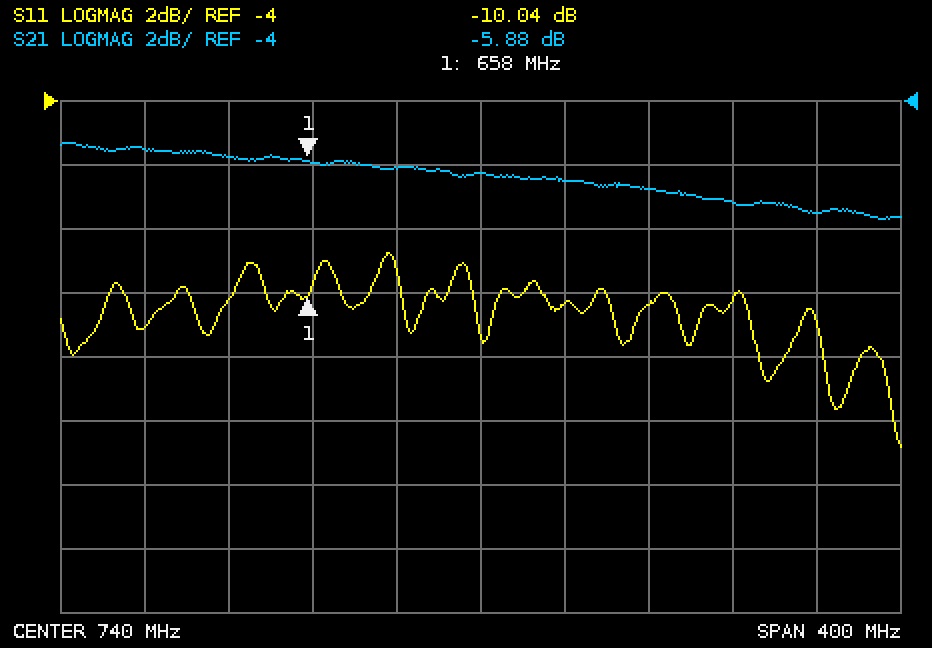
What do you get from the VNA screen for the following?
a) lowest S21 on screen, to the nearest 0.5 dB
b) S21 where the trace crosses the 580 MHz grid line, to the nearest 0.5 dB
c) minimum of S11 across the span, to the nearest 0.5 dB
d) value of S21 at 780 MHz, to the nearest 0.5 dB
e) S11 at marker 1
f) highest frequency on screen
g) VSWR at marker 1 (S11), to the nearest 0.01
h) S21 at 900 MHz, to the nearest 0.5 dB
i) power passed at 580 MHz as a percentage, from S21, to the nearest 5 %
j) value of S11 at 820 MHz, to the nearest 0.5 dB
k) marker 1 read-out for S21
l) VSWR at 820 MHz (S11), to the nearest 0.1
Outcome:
-7.5 dB
-5.5 dB
-15.0 dB
-6.5 dB
-10.04 dB
940 MHz
1.92
-7.5 dB
30 %
-10.5 dB
-5.88 dB
1.9
